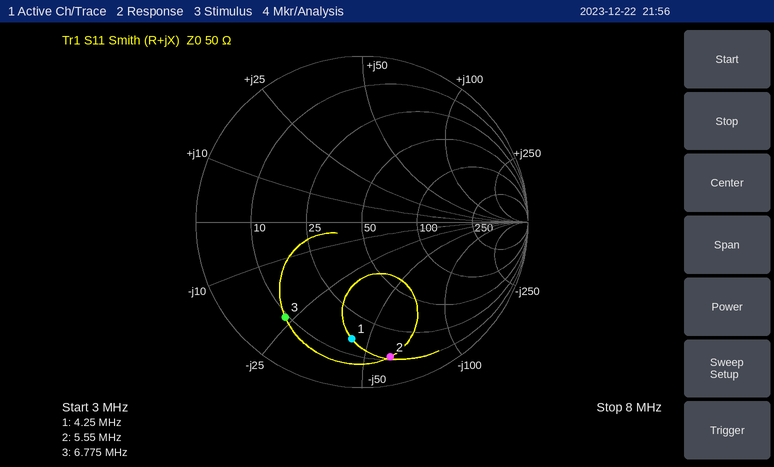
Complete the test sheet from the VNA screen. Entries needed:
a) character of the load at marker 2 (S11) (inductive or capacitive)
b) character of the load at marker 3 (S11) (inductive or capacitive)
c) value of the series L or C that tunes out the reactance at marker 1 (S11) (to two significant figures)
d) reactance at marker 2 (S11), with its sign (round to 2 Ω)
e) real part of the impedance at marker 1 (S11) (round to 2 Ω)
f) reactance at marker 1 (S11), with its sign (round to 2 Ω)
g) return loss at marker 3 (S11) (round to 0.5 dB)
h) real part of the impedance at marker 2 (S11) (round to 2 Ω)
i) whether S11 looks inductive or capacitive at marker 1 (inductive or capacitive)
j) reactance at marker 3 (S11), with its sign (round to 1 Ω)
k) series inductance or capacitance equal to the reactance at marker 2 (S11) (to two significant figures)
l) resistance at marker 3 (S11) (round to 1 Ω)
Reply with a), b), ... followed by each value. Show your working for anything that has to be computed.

a) capacitive
b) capacitive
c) L = 44 Ω/(2π × 4.25 MHz) ≈ 1.6 µH
d) -60 Ω
e) 16 Ω
f) -44 Ω
g) 2.5 dB
h) 12 Ω
i) capacitive
j) -23 Ω
k) C = 1/(2π × 5.55 MHz × 60 Ω) ≈ 478 pF, so 480 pF to two significant figures
l) 9 Ω
